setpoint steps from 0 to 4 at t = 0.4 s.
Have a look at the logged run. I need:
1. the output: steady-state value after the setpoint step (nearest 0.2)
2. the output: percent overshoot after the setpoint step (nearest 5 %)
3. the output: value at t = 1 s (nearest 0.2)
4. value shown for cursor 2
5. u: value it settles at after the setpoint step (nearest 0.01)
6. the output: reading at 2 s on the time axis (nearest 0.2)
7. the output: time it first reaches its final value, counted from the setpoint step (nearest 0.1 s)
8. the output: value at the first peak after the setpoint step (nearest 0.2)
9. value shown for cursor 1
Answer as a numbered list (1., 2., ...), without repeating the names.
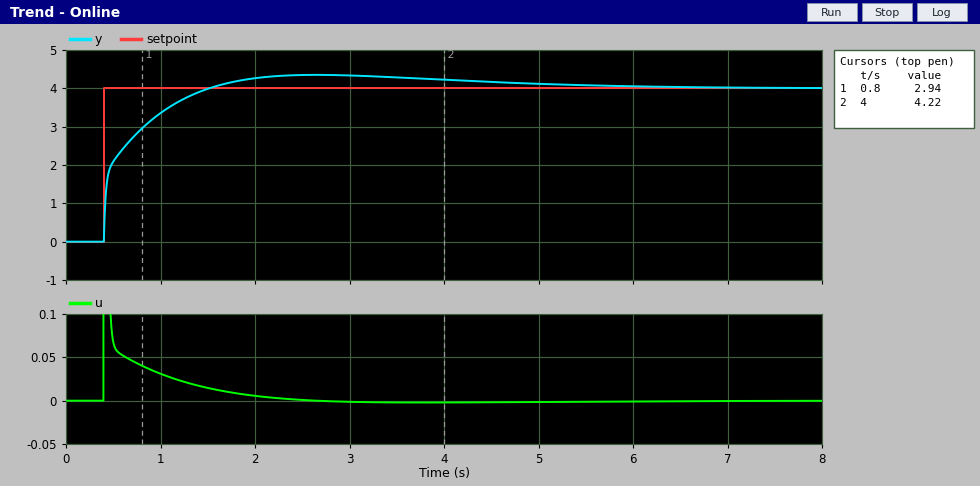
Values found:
1. 4.0
2. 10 %
3. 3.4
4. 4.22
5. 0.00
6. 4.2
7. 1.1 s
8. 4.4
9. 2.94
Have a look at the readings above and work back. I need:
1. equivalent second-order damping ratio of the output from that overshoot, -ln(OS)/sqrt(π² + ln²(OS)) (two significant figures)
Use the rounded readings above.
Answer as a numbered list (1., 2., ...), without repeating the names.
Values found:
1. 0.59
